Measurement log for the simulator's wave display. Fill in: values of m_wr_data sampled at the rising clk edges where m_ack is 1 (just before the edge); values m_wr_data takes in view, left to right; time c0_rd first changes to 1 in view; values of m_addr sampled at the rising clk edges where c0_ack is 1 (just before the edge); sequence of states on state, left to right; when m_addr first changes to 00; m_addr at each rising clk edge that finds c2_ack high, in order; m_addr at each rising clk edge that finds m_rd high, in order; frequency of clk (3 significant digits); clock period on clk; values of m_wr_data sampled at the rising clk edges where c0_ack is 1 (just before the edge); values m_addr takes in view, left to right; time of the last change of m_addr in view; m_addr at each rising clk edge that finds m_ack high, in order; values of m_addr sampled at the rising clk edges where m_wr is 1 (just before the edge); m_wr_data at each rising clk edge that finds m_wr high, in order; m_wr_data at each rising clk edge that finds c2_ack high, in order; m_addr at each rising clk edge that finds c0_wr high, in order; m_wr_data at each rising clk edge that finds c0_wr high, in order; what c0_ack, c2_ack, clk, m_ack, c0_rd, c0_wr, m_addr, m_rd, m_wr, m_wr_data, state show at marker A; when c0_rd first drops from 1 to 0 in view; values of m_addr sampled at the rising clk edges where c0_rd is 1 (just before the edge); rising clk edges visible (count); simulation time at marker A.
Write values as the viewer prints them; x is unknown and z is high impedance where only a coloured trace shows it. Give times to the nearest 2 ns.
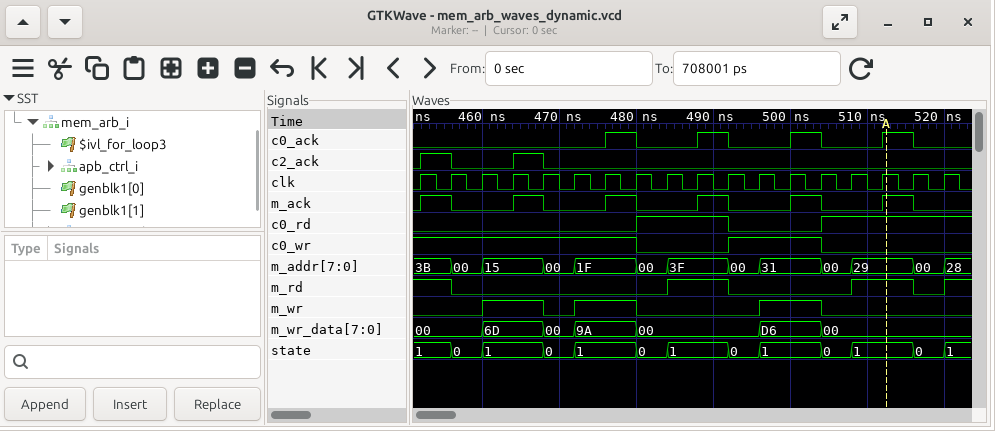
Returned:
00, 6D, 9A, 00, D6, 00
00, 6D, 00, 9A, 00, D6, 00
480 ns
1F, 3F, 31, 29
1, 0, 1, 0, 1, 0, 1, 0, 1, 0, 1, 0, 1
456 ns
3B, 15
3B, 3B, 3F, 3F, 29, 29
250 MHz
4 ns
9A, 00, D6, 00
3B, 00, 15, 00, 1F, 00, 3F, 00, 31, 00, 29, 00, 28
520 ns
3B, 15, 1F, 3F, 31, 29
15, 15, 1F, 1F, 31, 31
6D, 6D, 9A, 9A, D6, D6
00, 6D
3B, 3B, 00, 15, 15, 00, 1F, 1F, 00, 31, 31
00, 00, 00, 6D, 6D, 00, 9A, 9A, 00, D6, D6
c0_ack=1, c2_ack=0, clk=1, m_ack=1, c0_rd=1, c0_wr=0, m_addr=29, m_rd=1, m_wr=0, m_wr_data=00, state=1
492 ns
00, 3F, 3F, 00, 29, 29, 00
18
512 ns
